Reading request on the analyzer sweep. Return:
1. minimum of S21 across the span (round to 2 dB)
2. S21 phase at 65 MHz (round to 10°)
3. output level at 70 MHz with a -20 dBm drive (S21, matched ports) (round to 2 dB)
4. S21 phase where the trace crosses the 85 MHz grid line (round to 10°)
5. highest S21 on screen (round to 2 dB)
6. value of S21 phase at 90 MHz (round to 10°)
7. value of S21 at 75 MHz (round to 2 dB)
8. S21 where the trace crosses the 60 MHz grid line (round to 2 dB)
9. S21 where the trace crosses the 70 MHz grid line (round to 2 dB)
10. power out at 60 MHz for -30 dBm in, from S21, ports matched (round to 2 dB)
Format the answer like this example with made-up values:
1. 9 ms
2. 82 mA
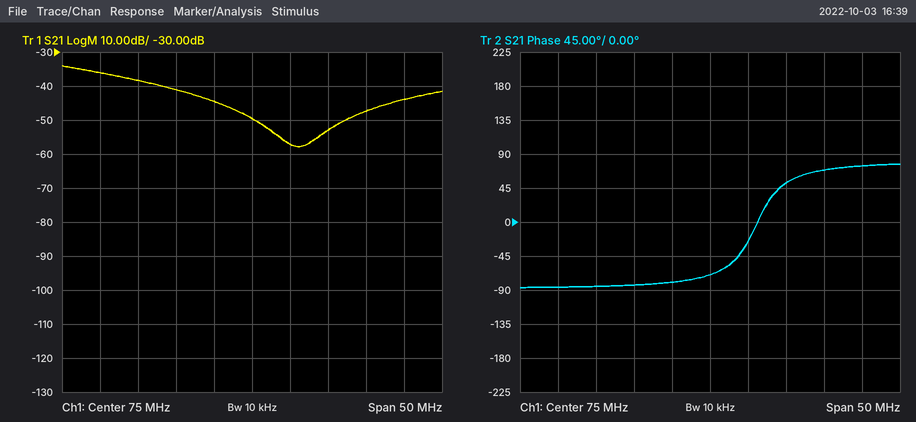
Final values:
1. -58 dB
2. -80°
3. -64 dBm
4. 50°
5. -34 dB
6. 70°
7. -50 dB
8. -38 dB
9. -44 dB
10. -68 dBm
